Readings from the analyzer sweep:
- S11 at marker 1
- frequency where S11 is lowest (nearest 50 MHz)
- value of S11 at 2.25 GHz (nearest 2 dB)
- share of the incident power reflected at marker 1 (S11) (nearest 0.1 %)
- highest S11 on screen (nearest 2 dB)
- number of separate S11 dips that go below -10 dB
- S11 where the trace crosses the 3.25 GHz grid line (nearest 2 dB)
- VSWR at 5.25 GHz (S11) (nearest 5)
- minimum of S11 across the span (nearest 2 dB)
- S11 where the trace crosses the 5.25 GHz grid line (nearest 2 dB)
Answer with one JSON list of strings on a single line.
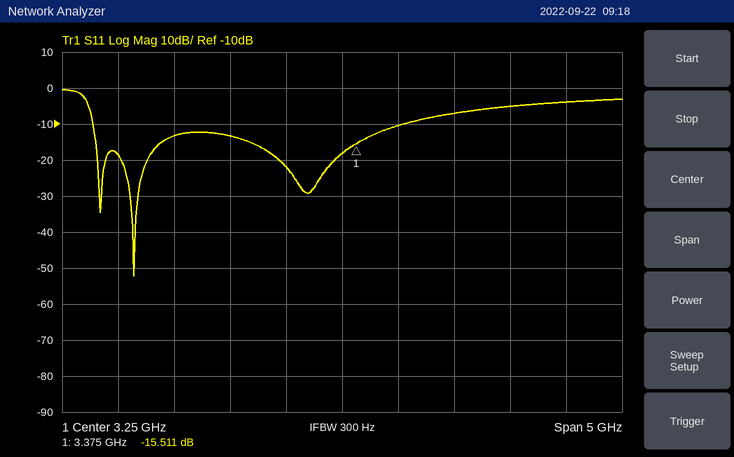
["-15.511 dB", "1.40 GHz", "-14 dB", "2.8 %", "0 dB", "3", "-18 dB", "5", "-52 dB", "-4 dB"]
